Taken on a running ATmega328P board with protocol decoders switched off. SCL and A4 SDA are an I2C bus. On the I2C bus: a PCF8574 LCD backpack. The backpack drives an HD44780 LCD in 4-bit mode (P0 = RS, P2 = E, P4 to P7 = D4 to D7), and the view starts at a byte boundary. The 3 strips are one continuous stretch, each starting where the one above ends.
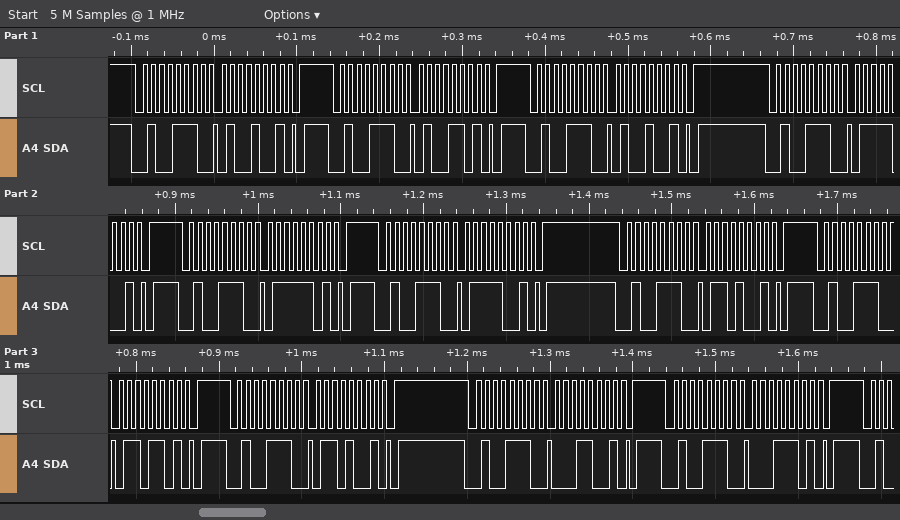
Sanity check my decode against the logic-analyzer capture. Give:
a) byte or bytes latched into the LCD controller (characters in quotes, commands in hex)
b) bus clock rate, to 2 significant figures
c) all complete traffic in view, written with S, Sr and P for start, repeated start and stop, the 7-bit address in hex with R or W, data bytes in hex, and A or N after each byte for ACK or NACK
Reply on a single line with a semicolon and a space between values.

'G'; 100 kHz; S 27W A 49 A P S 27W A 4D A P S 27W A 49 A P S 27W A 79 A P S 27W A 7D A P S 27W A 79 A P S 27W A 69 A P S 27W A 6D A P S 27W A 69 A P S 27W A 19 A P S 27W A 1D A P
